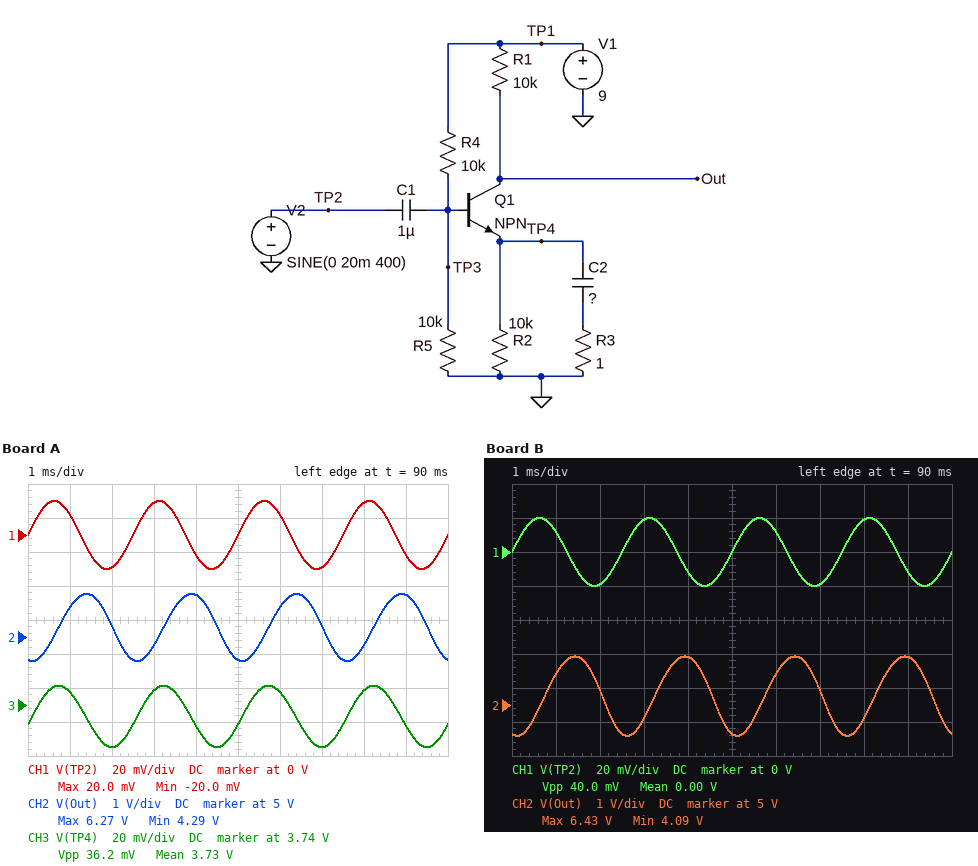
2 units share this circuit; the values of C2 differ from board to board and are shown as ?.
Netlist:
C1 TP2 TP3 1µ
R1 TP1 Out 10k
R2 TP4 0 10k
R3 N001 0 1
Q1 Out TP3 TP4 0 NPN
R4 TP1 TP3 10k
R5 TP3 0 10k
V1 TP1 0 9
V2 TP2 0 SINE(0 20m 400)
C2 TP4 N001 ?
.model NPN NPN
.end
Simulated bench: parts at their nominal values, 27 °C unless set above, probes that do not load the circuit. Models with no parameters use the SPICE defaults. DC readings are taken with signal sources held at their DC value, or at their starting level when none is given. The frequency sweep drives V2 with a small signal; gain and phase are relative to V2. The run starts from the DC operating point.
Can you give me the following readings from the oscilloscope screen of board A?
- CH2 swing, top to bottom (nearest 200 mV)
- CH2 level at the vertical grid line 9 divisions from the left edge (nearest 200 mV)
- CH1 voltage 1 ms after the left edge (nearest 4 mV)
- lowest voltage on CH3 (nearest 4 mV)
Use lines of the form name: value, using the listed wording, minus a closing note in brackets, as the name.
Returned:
CH2 swing, top to bottom: 2.0 V
CH2 level at the vertical grid line 9 divisions from the left edge: 6.2 V
CH1 voltage 1 ms after the left edge: 12 mV
lowest voltage on CH3: 3.716 V
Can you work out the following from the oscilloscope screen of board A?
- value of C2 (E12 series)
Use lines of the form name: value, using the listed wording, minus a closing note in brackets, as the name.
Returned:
value of C2: 2.2 µF
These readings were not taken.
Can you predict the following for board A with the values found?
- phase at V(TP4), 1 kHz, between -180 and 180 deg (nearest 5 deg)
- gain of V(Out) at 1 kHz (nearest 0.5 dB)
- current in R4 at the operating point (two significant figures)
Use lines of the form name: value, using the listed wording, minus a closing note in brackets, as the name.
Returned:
phase at V(TP4), 1 kHz, between -180 and 180 deg: -40 deg
gain of V(Out) at 1 kHz: 39.5 dB
current in R4 at the operating point: 450 µA
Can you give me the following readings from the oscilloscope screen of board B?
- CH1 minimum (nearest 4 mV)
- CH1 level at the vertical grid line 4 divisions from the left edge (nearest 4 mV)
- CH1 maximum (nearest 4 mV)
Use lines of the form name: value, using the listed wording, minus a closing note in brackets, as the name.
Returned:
CH1 minimum: -20 mV
CH1 level at the vertical grid line 4 divisions from the left edge: -12 mV
CH1 maximum: 20 mV
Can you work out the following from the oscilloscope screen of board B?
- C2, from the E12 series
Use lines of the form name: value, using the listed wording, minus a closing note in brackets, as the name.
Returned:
C2, from the E12 series: 2.7 µF
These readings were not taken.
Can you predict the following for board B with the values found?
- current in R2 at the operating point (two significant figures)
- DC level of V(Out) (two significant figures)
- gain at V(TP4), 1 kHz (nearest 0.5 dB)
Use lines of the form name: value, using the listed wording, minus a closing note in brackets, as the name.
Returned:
current in R2 at the operating point: 370 µA
DC level of V(Out): 5.3 V
gain at V(TP4), 1 kHz: -4.0 dB
